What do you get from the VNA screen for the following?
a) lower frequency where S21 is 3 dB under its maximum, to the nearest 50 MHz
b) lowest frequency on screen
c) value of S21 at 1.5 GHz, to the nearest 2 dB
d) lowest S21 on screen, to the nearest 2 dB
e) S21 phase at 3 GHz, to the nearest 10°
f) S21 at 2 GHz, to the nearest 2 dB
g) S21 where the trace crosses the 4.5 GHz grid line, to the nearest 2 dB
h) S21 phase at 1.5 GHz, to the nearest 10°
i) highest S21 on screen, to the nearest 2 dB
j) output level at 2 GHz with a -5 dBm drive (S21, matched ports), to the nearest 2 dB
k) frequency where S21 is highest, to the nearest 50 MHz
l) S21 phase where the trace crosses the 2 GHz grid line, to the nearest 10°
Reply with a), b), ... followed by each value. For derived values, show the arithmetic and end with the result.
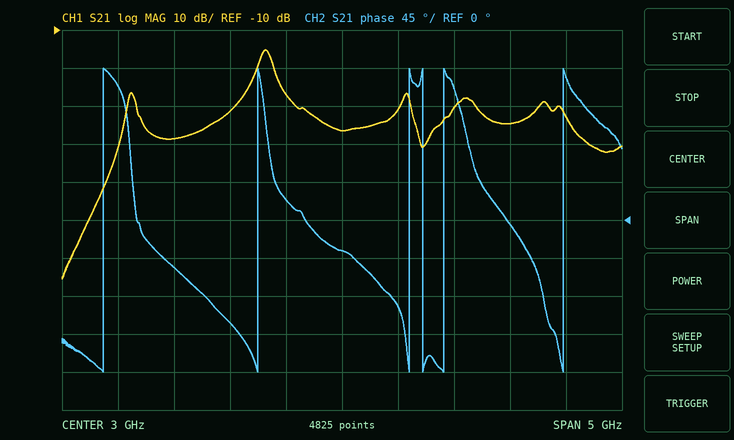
a) 2.25 GHz
b) 500 MHz
c) -38 dB
d) -76 dB
e) -40°
f) -32 dB
g) -34 dB
h) -60°
i) -16 dB
j) -5 dBm + (-32 dB) = -36 dBm
k) 2.30 GHz
l) -120°
